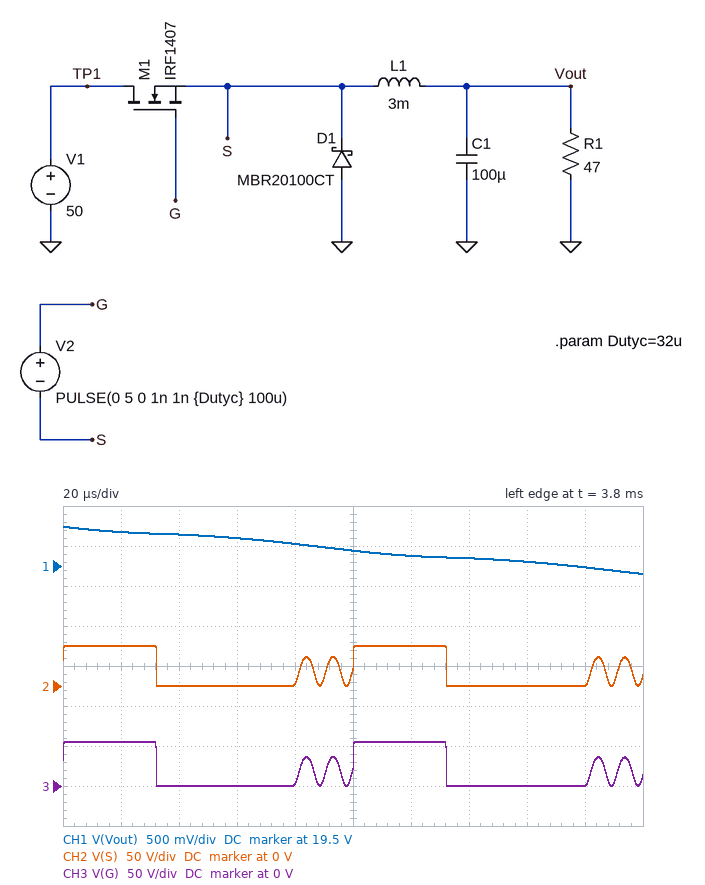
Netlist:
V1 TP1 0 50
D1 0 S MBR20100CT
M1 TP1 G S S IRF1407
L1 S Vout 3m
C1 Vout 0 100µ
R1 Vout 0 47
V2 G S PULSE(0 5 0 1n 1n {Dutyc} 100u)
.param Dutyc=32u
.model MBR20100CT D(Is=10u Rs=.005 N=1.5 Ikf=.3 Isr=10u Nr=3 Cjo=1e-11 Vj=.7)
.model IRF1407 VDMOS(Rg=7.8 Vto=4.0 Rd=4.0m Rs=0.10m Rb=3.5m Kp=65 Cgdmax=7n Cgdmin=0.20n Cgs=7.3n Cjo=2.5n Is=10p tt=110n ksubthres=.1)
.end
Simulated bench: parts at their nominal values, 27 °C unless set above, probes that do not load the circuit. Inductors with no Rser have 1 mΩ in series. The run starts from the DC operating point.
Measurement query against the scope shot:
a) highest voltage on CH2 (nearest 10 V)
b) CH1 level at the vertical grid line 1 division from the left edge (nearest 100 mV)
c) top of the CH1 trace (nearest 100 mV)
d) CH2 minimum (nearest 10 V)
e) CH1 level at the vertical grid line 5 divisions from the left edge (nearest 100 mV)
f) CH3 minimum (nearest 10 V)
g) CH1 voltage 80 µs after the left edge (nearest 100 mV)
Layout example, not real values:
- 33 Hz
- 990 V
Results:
- 50 V
- 19.9 V
- 20.0 V
- 0 V
- 19.7 V
- 0 V
- 19.8 V
